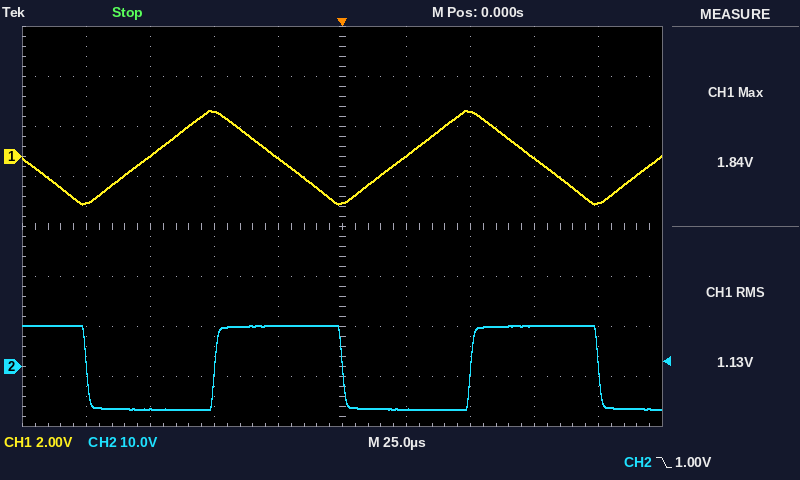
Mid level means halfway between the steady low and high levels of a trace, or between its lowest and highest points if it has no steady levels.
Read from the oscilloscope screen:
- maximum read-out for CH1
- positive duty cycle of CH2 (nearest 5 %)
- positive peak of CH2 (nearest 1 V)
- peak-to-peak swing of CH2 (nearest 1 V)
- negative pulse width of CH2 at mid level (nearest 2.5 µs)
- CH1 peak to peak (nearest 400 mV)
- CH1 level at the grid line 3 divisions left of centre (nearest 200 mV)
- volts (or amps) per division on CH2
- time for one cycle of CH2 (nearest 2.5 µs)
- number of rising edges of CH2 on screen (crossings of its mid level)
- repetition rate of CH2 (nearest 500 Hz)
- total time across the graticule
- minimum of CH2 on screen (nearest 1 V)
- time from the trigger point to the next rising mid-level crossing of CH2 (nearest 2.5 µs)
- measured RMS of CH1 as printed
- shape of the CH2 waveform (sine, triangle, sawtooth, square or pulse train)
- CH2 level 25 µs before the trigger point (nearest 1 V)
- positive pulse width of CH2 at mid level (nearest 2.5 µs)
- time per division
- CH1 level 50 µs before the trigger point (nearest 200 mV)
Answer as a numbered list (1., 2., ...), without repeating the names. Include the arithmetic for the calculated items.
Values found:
1. 1.84 V
2. 50.0 µs / 100.0 µs ≈ 50 %
3. 8 V
4. 8 V − (-9 V) = 17 V
5. 50.0 µs
6. 3.6 V
7. 0.0 V
8. 10 V
9. 100.0 µs
10. 2
11. 1 / 100.0 µs ≈ 10.0 kHz
12. 250 µs
13. -9 V
14. 50.0 µs
15. 1.13 V
16. square
17. 8 V
18. 50.0 µs
19. 25 µs
20. 1.8 V
